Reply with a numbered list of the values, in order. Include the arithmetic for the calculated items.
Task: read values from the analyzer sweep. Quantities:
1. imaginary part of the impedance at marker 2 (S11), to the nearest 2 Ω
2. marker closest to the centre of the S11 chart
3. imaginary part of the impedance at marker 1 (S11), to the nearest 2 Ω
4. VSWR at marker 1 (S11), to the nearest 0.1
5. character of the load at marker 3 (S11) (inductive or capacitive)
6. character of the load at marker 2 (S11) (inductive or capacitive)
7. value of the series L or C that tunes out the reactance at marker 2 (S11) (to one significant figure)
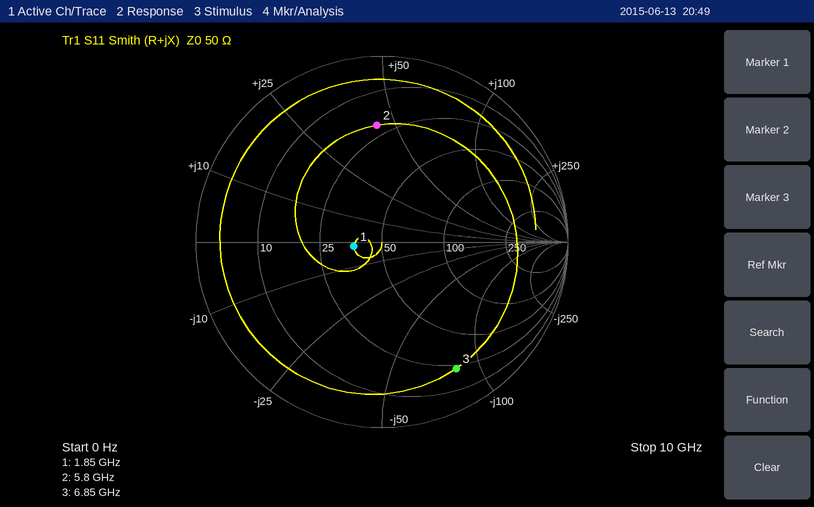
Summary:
1. +44 Ω
2. marker 1
3. -2 Ω
4. 1.4
5. capacitive
6. inductive
7. C = 1/(2π × 5.8 GHz × 44 Ω) ≈ 624 fF, so 600 fF to one significant figure
